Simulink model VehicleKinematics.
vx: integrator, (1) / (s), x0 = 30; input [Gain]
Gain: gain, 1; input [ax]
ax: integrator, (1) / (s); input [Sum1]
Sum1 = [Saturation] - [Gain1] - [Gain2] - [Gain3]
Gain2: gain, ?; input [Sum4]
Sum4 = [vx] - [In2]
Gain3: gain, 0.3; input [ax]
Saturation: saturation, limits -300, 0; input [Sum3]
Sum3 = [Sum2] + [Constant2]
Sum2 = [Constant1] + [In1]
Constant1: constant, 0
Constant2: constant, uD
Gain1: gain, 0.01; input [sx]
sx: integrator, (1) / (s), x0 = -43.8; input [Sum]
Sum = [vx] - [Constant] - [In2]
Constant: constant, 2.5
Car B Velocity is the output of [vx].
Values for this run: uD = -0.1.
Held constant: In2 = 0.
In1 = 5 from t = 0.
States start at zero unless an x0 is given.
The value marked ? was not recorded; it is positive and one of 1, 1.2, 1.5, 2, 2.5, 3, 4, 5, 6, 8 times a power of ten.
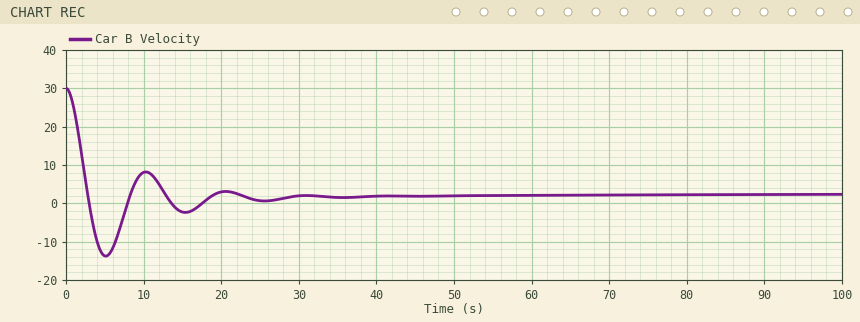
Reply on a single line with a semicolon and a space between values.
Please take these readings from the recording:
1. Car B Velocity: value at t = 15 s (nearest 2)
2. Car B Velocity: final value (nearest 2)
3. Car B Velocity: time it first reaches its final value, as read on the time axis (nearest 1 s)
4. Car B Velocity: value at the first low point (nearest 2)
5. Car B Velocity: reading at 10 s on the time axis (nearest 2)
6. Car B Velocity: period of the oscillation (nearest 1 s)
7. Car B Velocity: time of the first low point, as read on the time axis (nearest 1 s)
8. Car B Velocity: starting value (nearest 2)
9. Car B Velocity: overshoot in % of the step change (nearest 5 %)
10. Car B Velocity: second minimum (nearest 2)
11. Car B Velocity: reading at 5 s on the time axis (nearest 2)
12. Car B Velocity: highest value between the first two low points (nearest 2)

-2; 2; 3 s; -14; 8; 10 s; 5 s; 30; 60 %; -2; -14; 8
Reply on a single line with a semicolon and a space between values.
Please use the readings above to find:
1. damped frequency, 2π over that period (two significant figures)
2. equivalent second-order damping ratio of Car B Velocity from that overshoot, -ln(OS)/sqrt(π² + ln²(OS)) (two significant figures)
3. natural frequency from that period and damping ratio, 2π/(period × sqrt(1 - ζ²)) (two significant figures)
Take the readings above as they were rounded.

0.63 rad/s; 0.16; 0.64 rad/s
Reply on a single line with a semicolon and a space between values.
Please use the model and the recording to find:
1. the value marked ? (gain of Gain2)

0.4
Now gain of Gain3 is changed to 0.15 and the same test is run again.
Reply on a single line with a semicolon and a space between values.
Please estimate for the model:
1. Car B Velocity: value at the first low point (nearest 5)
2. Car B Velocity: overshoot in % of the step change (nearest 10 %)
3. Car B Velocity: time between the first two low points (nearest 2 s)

-20; 80 %; 10 s
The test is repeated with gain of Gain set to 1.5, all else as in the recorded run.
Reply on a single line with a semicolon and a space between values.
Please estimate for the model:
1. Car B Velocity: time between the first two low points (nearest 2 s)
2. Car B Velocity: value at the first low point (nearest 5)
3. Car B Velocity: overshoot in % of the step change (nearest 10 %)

8 s; -15; 70 %
